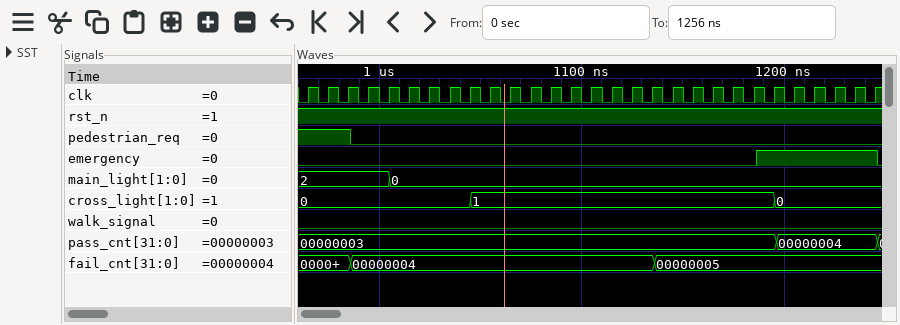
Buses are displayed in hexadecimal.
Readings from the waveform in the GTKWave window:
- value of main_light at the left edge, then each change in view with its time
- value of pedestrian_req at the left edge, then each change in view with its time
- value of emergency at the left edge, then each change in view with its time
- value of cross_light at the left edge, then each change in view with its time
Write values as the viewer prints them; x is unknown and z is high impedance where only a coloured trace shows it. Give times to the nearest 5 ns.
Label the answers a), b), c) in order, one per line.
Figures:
a) 2, 0 at 1005 ns
b) 1, 0 at 985 ns
c) 0, 1 at 1185 ns, 0 at 1245 ns
d) 0, 1 at 1045 ns, 0 at 1195 ns
